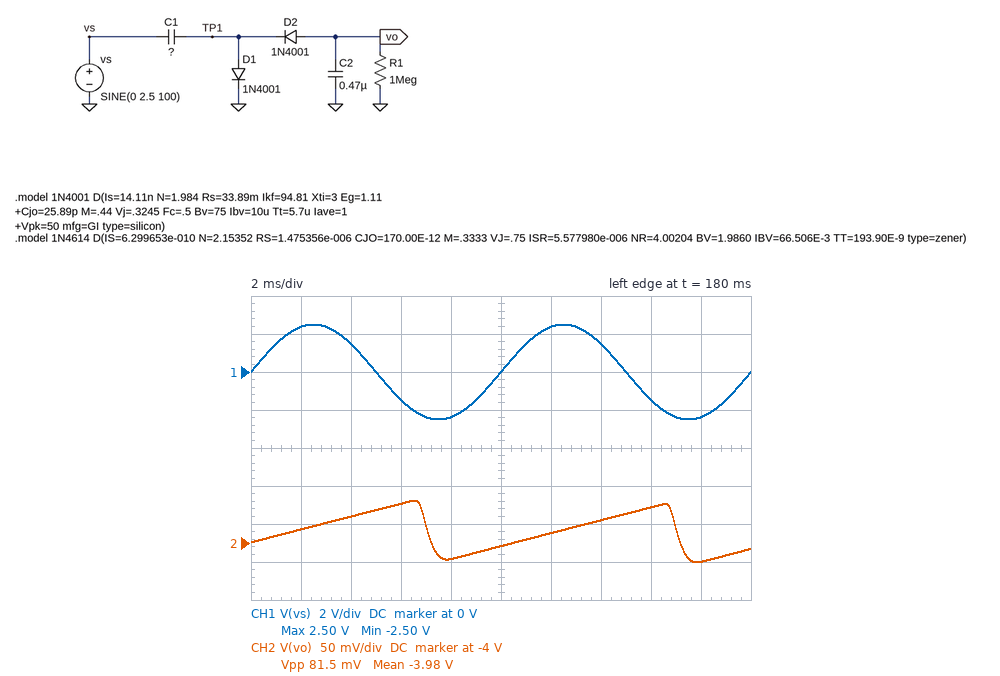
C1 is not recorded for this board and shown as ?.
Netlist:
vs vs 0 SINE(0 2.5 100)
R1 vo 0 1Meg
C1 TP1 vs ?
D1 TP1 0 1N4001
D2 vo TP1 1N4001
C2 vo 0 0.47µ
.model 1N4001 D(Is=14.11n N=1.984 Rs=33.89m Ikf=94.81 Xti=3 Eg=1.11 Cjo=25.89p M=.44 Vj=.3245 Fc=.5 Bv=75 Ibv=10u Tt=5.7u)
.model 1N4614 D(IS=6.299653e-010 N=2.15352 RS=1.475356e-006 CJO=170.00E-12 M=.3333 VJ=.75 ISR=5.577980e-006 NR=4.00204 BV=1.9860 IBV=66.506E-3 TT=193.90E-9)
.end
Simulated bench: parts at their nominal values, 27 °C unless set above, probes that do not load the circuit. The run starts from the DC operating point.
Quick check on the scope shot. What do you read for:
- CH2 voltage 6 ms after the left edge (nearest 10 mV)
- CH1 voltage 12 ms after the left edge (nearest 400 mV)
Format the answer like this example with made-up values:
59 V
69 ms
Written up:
-3.95 V
2.4 V
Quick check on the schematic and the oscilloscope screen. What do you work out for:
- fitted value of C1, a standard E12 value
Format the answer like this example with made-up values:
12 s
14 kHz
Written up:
150 nF
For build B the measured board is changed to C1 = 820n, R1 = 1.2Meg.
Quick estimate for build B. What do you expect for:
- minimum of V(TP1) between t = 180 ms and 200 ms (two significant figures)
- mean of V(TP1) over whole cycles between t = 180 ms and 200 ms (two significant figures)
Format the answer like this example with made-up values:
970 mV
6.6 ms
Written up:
-4.6 V
-2.1 V
